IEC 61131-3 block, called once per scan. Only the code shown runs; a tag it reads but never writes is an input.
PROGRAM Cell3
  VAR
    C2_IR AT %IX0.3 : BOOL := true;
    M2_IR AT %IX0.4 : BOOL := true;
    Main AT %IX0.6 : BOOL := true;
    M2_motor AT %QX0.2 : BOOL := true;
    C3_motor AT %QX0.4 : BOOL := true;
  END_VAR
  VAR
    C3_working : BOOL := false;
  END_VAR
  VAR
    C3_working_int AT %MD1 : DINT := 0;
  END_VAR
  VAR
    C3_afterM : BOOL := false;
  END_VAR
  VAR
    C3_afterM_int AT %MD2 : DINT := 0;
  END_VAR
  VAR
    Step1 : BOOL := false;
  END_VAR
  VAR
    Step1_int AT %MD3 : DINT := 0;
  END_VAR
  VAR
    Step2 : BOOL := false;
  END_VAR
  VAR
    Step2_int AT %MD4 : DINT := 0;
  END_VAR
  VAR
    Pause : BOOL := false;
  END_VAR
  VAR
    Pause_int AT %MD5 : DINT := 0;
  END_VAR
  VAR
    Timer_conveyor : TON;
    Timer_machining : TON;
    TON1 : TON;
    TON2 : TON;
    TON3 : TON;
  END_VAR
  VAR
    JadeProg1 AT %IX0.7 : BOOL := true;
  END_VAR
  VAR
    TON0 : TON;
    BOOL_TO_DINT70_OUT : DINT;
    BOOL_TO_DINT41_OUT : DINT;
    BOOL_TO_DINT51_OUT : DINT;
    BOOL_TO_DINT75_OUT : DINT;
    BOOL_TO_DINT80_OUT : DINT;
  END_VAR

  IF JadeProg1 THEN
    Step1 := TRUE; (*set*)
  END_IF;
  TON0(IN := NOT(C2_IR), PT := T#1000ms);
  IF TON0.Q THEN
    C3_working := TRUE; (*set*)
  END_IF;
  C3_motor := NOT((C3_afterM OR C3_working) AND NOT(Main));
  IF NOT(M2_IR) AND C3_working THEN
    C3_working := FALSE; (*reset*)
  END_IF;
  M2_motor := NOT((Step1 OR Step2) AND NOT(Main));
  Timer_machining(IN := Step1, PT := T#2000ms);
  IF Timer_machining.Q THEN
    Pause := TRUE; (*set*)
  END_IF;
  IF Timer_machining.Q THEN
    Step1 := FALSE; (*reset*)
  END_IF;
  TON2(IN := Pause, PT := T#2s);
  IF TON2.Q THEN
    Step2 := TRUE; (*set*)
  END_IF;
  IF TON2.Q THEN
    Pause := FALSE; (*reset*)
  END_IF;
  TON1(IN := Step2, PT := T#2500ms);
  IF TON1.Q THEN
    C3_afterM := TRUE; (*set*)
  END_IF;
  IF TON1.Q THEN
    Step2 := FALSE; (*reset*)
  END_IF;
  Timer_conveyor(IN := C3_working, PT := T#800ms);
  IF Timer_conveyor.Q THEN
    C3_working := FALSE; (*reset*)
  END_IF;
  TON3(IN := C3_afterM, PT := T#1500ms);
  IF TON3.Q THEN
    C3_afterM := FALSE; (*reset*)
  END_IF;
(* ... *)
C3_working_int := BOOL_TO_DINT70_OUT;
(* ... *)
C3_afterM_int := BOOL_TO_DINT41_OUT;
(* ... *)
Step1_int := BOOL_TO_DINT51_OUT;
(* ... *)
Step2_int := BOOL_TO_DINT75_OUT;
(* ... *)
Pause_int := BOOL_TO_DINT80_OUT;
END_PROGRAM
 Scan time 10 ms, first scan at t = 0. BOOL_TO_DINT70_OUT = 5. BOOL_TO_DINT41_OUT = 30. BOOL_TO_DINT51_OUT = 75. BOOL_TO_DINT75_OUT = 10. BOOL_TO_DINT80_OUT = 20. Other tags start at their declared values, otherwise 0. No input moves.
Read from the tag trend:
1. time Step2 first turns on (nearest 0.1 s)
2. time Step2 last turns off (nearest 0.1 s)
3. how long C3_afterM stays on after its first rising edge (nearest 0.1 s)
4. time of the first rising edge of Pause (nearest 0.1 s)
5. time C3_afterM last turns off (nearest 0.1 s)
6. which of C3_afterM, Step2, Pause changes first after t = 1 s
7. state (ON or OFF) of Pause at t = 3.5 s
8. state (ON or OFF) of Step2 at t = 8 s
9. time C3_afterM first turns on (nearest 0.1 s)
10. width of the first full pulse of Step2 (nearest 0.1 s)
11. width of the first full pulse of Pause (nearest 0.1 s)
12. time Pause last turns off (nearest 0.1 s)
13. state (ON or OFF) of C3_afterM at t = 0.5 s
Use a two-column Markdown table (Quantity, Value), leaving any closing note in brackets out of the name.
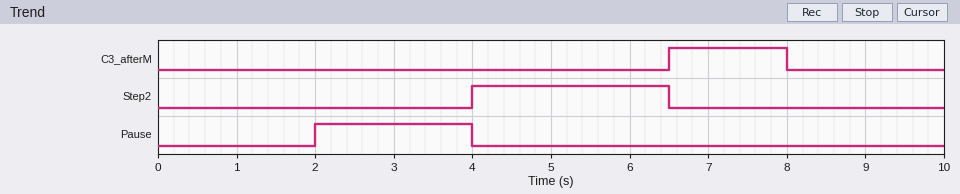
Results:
| Quantity | Value |
|---|---|
| time Step2 first turns on | 4.0 s |
| time Step2 last turns off | 6.5 s |
| how long C3_afterM stays on after its first rising edge | 1.5 s |
| time of the first rising edge of Pause | 2.0 s |
| time C3_afterM last turns off | 8.0 s |
| which of C3_afterM, Step2, Pause changes first after t = 1 s | Pause |
| state (ON or OFF) of Pause at t = 3.5 s | ON |
| state (ON or OFF) of Step2 at t = 8 s | OFF |
| time C3_afterM first turns on | 6.5 s |
| width of the first full pulse of Step2 | 2.5 s |
| width of the first full pulse of Pause | 2.0 s |
| time Pause last turns off | 4.0 s |
| state (ON or OFF) of C3_afterM at t = 0.5 s | OFF |
